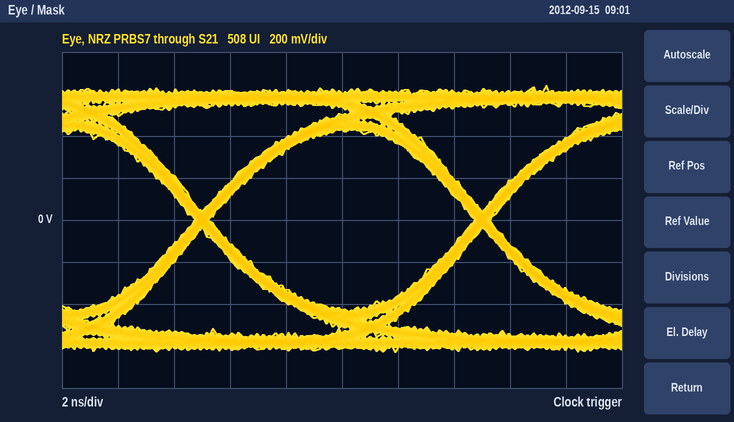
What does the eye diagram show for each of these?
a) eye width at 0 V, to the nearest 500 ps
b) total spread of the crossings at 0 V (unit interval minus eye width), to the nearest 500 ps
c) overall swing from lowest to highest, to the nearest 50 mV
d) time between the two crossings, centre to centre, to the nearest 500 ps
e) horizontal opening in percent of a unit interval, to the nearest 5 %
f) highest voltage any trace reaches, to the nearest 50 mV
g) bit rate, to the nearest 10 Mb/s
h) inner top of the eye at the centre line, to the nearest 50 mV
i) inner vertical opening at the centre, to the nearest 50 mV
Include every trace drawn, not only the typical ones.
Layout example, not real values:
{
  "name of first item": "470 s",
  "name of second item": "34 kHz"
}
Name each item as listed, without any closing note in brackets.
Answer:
{
  "eye width at 0 V, to the nearest 500 ps": "9.5 ns",
  "total spread of the crossings at 0 V (unit interval minus eye width), to the nearest 500 ps": "500 ps",
  "overall swing from lowest to highest, to the nearest 50 mV": "1.25 V",
  "time between the two crossings, centre to centre, to the nearest 500 ps": "10.0 ns",
  "horizontal opening in percent of a unit interval, to the nearest 5 %": "95 %",
  "highest voltage any trace reaches, to the nearest 50 mV": "650 mV",
  "bit rate, to the nearest 10 Mb/s": "100 Mb/s",
  "inner top of the eye at the centre line, to the nearest 50 mV": "450 mV",
  "inner vertical opening at the centre, to the nearest 50 mV": "850 mV"
}
